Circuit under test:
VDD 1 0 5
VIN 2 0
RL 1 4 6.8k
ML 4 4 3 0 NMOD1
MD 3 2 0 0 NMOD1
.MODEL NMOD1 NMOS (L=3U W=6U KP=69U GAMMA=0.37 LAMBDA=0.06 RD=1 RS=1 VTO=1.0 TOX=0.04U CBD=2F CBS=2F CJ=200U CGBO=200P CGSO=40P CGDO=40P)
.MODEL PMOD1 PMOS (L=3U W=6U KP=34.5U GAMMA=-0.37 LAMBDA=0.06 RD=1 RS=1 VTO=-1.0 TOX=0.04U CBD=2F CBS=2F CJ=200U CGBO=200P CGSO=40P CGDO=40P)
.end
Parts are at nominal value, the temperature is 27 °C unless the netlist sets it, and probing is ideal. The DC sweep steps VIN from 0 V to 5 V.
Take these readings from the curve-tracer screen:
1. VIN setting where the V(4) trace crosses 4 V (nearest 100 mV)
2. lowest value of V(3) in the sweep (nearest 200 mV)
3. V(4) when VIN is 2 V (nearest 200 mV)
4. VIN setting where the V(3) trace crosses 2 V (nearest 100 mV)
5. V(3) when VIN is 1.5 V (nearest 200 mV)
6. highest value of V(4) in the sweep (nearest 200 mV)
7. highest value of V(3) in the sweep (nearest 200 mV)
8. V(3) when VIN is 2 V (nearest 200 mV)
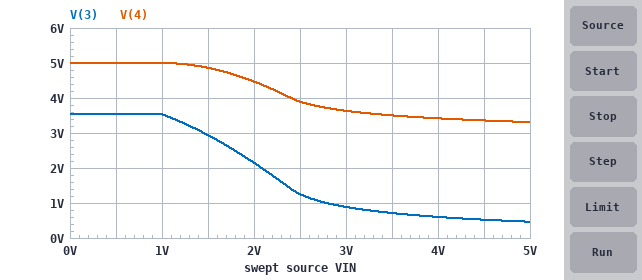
2.4 V
400 mV
4.4 V
2.1 V
3.0 V
5.0 V
3.6 V
2.2 V
